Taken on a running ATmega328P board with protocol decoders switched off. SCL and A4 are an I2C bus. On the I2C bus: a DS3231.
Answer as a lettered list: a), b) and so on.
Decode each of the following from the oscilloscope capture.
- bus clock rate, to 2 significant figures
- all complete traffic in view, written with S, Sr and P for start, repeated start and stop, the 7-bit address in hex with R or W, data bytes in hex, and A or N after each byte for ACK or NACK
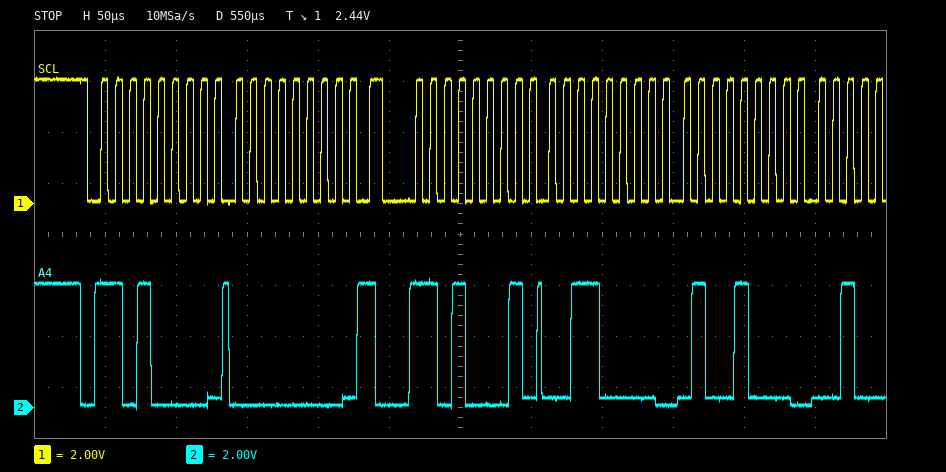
a) 100 kHz
b) S 68W A 00 A Sr 68R A 30 A 48 A
